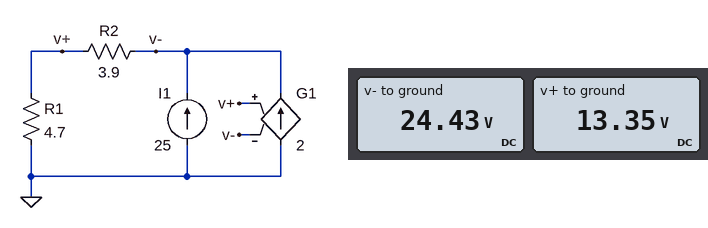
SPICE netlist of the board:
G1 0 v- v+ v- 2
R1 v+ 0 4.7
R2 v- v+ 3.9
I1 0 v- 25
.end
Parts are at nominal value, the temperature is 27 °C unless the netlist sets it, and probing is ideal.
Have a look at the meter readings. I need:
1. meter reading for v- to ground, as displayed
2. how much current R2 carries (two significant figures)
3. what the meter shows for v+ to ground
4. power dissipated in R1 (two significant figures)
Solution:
24.43 V
2.8 A
13.35 V
38 W
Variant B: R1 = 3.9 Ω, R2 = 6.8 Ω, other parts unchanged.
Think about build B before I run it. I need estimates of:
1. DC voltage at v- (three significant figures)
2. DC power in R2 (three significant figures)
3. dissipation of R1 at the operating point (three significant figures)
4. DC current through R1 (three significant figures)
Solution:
18.3 V
19.9 W
11.4 W
1.71 A
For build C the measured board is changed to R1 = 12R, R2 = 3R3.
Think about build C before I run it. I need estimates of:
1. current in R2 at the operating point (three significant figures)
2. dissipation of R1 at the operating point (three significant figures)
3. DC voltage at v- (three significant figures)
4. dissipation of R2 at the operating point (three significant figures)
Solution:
3.29 A
130 W
50.3 V
35.7 W
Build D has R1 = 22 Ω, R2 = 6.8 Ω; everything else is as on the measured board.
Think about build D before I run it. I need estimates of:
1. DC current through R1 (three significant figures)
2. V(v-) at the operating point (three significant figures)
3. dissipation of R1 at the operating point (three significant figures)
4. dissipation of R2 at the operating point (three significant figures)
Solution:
1.71 A
49.3 V
64.5 W
19.9 W
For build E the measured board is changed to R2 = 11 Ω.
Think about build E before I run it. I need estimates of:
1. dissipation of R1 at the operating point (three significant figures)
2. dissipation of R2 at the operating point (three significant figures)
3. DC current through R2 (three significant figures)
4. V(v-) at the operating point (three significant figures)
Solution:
5.55 W
13.0 W
1.09 A
17.1 V
